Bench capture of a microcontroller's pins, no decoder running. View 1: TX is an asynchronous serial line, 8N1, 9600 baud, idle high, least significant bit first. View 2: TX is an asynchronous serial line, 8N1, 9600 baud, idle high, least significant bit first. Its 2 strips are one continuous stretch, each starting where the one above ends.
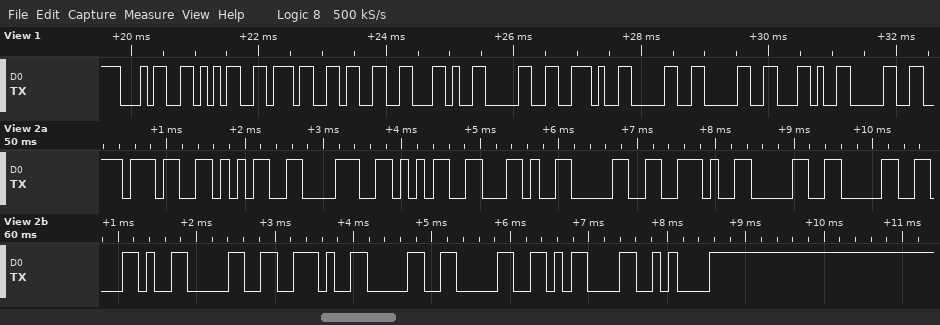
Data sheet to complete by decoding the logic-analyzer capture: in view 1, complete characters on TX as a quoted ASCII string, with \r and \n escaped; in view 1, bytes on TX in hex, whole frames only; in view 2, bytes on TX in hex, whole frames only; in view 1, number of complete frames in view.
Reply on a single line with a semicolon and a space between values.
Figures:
"4573,0.00,0"; 34 35 37 33 2C 30 2E 30 30 2C 30; 37 35 38 35 2C 30 2E 30 30 2C 30 2E 30 30 0D 0A; 11
